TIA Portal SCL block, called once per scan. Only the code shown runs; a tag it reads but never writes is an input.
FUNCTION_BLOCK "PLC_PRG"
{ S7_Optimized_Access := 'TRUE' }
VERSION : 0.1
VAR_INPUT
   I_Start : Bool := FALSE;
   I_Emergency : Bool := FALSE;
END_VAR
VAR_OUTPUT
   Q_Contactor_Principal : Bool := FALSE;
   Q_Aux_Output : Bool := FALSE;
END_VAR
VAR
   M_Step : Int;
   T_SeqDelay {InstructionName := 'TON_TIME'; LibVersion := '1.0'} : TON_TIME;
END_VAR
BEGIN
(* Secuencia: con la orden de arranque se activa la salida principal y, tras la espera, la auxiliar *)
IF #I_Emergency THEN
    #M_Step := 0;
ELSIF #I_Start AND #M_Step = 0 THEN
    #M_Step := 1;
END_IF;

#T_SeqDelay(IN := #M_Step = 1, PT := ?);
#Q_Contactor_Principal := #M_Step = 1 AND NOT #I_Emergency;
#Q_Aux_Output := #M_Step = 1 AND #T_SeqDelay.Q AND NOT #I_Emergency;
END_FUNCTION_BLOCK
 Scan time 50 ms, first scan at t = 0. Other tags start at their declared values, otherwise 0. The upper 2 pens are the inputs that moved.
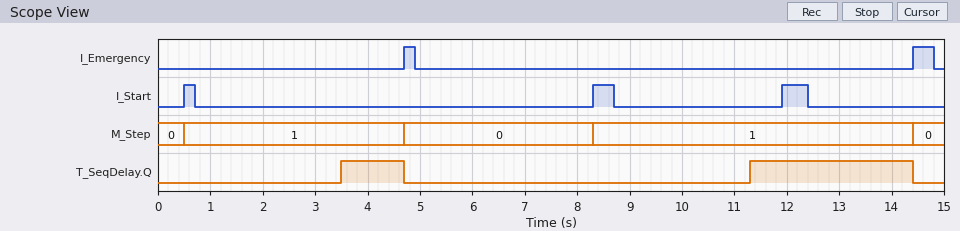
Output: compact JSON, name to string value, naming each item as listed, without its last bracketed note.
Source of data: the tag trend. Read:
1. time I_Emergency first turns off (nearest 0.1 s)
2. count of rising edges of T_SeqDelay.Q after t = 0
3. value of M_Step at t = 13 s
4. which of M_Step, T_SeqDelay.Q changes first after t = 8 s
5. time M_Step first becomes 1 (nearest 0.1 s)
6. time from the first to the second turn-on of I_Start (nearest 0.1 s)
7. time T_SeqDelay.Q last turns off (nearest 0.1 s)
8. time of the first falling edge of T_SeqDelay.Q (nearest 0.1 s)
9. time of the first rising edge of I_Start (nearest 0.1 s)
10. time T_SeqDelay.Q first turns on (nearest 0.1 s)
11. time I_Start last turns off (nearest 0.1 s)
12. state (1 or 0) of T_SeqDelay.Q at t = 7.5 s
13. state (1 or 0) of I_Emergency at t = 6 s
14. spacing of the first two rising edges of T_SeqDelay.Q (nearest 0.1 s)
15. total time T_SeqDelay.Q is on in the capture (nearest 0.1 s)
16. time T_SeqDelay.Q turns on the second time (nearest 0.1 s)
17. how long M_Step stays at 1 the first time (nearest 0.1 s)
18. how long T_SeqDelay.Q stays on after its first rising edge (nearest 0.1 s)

{"time I_Emergency first turns off": "4.9 s", "count of rising edges of T_SeqDelay.Q after t = 0": "2", "value of M_Step at t = 13 s": "1", "which of M_Step, T_SeqDelay.Q changes first after t = 8 s": "M_Step", "time M_Step first becomes 1": "0.5 s", "time from the first to the second turn-on of I_Start": "7.8 s", "time T_SeqDelay.Q last turns off": "14.4 s", "time of the first falling edge of T_SeqDelay.Q": "4.7 s", "time of the first rising edge of I_Start": "0.5 s", "time T_SeqDelay.Q first turns on": "3.5 s", "time I_Start last turns off": "12.4 s", "state (1 or 0) of T_SeqDelay.Q at t = 7.5 s": "0", "state (1 or 0) of I_Emergency at t = 6 s": "0", "spacing of the first two rising edges of T_SeqDelay.Q": "7.8 s", "total time T_SeqDelay.Q is on in the capture": "4.3 s", "time T_SeqDelay.Q turns on the second time": "11.3 s", "how long M_Step stays at 1 the first time": "4.2 s", "how long T_SeqDelay.Q stays on after its first rising edge": "1.2 s"}
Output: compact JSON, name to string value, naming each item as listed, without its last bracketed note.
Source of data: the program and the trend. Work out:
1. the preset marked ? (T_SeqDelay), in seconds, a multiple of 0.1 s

{"the preset marked ? (T_SeqDelay), in seconds, a multiple of 0.1 s": "3.0 s"}
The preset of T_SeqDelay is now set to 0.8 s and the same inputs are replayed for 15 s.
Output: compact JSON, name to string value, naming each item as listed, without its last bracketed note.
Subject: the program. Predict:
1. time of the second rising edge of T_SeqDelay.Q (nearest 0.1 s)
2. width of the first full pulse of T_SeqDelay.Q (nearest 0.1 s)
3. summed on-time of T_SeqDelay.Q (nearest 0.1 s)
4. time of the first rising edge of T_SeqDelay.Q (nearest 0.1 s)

{"time of the second rising edge of T_SeqDelay.Q": "9.1 s", "width of the first full pulse of T_SeqDelay.Q": "3.4 s", "summed on-time of T_SeqDelay.Q": "8.7 s", "time of the first rising edge of T_SeqDelay.Q": "1.3 s"}
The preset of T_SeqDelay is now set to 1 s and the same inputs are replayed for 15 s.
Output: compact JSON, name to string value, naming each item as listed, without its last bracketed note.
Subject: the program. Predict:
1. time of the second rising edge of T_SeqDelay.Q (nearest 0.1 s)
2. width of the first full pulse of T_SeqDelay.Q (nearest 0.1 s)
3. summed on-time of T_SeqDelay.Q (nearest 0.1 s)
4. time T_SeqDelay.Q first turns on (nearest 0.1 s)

{"time of the second rising edge of T_SeqDelay.Q": "9.3 s", "width of the first full pulse of T_SeqDelay.Q": "3.2 s", "summed on-time of T_SeqDelay.Q": "8.3 s", "time T_SeqDelay.Q first turns on": "1.5 s"}
